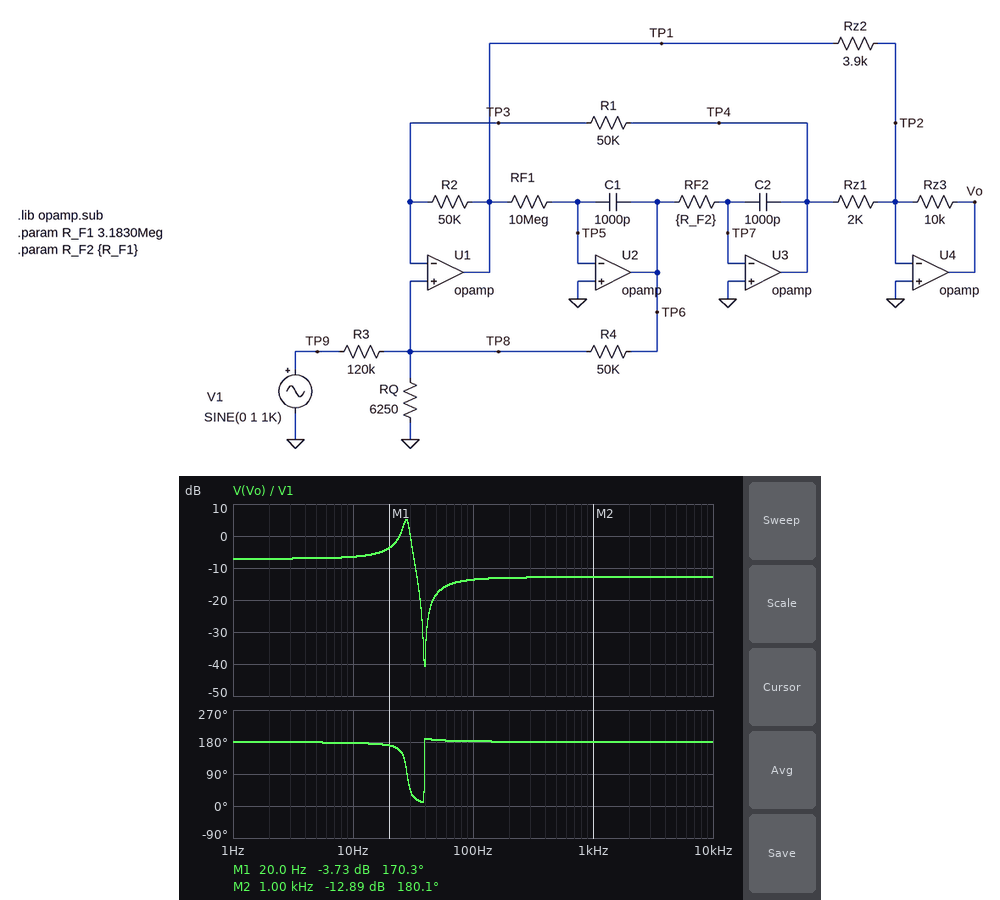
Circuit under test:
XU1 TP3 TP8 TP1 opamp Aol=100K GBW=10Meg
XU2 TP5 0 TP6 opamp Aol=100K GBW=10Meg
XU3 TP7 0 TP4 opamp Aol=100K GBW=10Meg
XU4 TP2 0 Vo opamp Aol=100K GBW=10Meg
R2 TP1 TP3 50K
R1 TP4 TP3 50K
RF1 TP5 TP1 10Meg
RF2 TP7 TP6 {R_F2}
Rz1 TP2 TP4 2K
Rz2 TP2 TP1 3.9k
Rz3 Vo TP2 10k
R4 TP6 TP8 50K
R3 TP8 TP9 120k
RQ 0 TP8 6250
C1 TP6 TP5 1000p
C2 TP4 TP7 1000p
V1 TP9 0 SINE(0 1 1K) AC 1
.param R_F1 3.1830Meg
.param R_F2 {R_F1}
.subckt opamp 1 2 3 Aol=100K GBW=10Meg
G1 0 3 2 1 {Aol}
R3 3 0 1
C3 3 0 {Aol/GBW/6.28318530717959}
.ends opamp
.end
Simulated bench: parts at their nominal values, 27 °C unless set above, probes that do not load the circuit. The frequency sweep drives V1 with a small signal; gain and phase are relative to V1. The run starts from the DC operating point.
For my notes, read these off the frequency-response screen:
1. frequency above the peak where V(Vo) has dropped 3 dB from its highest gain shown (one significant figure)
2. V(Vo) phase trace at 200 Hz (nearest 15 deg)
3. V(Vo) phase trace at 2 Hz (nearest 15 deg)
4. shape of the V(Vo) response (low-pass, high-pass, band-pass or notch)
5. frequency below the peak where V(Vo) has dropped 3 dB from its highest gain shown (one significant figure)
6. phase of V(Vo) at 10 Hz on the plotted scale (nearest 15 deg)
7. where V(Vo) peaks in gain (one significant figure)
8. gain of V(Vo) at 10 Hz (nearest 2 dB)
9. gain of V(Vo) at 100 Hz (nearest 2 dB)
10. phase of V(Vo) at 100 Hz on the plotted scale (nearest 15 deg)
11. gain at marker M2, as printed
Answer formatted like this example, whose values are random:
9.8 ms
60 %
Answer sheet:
30 Hz
180 deg
180 deg
band-pass
30 Hz
180 deg
30 Hz
-6 dB
-14 dB
180 deg
-12.89 dB
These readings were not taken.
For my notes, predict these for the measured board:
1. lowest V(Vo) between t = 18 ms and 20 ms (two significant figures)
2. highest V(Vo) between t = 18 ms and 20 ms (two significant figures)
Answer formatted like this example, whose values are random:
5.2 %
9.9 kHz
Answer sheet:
-230 mV
230 mV
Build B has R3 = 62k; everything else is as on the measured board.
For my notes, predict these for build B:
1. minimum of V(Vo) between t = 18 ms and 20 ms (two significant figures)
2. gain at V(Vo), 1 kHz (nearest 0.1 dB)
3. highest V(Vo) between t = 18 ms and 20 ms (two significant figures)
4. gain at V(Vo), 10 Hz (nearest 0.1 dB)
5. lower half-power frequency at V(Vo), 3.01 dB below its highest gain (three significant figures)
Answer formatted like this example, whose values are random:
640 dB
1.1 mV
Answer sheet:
-420 mV
-7.5 dB
420 mV
-1.1 dB
26.0 Hz
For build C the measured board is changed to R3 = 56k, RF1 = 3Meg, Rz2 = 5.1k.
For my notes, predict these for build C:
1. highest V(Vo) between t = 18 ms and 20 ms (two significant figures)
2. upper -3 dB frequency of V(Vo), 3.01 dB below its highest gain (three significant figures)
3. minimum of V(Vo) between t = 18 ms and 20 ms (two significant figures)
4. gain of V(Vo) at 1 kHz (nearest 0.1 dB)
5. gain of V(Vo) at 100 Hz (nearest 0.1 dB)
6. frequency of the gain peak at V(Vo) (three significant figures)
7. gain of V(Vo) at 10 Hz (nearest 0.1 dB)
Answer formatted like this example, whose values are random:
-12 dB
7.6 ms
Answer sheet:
360 mV
54.9 Hz
-350 mV
-9.1 dB
-16.2 dB
50.2 Hz
-0.7 dB
